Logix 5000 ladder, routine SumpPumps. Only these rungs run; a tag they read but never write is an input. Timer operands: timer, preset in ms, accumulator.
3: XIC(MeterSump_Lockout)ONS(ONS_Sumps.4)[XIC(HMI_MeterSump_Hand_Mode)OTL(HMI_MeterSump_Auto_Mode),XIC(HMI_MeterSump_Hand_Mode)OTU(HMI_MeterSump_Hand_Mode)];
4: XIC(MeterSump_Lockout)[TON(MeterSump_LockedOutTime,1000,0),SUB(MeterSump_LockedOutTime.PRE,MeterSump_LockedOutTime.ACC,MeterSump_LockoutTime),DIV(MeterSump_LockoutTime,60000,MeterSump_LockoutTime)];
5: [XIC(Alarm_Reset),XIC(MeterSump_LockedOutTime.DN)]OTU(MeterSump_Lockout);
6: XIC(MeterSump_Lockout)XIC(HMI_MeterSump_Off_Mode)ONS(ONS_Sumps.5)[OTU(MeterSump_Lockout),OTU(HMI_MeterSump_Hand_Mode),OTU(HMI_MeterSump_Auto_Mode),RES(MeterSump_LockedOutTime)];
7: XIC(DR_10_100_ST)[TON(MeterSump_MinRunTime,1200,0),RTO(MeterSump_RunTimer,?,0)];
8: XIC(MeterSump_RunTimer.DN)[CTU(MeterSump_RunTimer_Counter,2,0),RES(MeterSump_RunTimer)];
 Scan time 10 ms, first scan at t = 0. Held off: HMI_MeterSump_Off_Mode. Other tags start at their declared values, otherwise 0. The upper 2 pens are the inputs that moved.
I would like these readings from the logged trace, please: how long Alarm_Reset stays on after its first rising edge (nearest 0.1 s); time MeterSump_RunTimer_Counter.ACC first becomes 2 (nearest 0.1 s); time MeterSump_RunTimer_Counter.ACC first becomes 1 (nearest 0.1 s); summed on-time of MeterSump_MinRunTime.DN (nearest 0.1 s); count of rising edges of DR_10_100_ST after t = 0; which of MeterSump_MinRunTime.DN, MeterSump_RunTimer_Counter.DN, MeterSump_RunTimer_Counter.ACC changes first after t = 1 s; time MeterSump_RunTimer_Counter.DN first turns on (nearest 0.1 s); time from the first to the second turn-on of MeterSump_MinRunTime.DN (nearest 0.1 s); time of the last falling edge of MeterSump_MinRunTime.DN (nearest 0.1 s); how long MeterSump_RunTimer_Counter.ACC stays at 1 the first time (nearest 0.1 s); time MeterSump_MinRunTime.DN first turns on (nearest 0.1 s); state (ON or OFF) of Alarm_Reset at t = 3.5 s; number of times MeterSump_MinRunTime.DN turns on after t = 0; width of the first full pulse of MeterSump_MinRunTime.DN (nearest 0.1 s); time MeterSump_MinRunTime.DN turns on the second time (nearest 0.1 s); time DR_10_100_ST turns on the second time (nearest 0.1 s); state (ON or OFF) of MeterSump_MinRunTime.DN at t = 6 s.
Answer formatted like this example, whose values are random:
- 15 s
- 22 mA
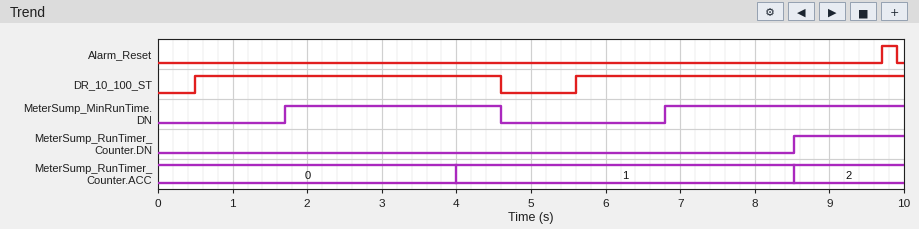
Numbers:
- 0.2 s
- 8.5 s
- 4.0 s
- 6.1 s
- 2
- MeterSump_MinRunTime.DN
- 8.5 s
- 5.1 s
- 4.6 s
- 4.5 s
- 1.7 s
- OFF
- 2
- 2.9 s
- 6.8 s
- 5.6 s
- OFF
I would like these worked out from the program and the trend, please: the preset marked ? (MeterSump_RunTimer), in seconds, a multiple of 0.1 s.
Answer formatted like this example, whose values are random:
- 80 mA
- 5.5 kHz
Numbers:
- 3.5 s
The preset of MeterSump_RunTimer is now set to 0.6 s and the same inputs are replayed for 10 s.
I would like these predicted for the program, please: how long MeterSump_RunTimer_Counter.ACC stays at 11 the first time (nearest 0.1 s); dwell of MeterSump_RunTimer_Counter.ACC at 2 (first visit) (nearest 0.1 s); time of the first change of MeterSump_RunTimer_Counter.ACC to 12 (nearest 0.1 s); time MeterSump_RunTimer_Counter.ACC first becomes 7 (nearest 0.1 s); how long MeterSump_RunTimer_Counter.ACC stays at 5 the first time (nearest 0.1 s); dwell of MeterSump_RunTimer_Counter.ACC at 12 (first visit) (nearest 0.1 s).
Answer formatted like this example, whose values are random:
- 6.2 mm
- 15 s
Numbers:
- 0.6 s
- 0.6 s
- 8.8 s
- 5.8 s
- 0.6 s
- 0.6 s
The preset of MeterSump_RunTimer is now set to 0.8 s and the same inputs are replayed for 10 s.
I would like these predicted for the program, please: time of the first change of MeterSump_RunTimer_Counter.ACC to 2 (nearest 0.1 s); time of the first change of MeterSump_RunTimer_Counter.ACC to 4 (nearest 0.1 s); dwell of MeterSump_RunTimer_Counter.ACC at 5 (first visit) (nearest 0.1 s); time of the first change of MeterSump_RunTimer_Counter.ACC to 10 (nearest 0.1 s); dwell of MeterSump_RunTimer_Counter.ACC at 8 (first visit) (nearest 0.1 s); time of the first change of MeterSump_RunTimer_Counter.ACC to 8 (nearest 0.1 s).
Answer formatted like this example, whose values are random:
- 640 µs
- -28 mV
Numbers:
- 2.1 s
- 3.7 s
- 1.8 s
- 9.6 s
- 0.8 s
- 8.0 s
